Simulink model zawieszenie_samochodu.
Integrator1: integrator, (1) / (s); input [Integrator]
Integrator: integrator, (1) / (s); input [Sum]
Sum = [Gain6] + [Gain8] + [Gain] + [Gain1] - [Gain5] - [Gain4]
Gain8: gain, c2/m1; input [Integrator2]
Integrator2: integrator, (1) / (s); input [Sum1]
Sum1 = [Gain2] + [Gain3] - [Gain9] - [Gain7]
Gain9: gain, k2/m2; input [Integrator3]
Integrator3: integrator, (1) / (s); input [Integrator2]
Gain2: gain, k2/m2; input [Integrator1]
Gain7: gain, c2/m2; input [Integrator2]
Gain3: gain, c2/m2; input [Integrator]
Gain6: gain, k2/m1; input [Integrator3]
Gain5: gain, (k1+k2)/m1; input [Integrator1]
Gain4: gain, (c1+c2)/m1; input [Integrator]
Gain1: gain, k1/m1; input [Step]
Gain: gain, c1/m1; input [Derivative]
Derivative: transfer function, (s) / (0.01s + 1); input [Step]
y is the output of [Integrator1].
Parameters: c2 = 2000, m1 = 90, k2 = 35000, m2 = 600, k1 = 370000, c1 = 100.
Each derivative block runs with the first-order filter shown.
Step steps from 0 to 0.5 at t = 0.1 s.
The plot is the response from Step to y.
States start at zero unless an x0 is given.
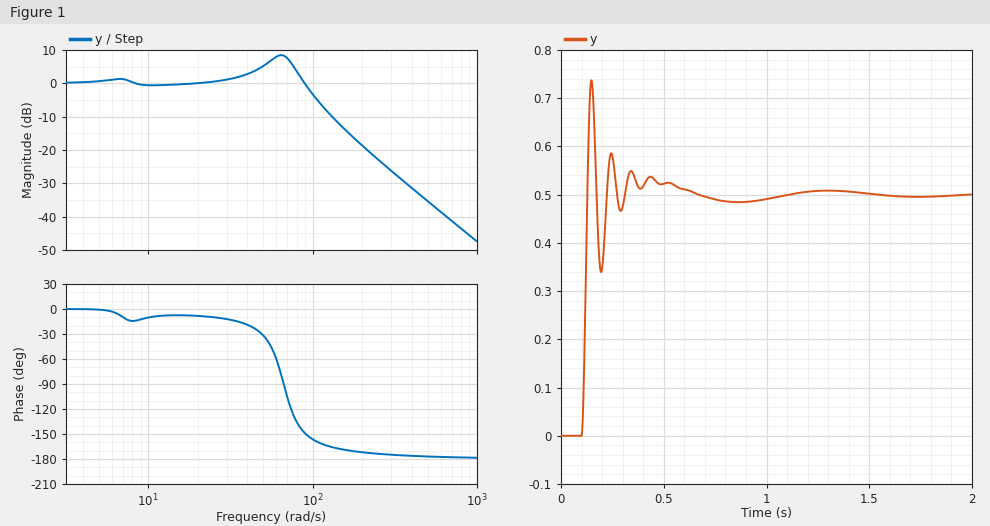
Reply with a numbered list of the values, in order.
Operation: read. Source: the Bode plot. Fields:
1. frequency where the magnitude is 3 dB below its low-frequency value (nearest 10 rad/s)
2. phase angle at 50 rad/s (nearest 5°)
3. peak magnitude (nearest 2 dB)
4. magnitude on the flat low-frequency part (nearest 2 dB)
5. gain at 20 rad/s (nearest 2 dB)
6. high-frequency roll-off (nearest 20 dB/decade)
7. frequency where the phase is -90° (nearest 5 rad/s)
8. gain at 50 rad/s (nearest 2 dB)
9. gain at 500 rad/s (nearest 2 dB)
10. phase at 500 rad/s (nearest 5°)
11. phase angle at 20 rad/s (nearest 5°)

1. 100 rad/s
2. -30°
3. 8 dB
4. 0 dB
5. 0 dB
6. -40 dB/decade
7. 65 rad/s
8. 6 dB
9. -36 dB
10. -175°
11. -10°
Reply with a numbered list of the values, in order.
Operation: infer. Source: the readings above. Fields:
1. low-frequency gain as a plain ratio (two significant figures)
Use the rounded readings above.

1. 1.0
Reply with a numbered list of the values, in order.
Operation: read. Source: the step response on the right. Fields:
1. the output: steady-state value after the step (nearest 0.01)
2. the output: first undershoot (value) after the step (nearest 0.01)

1. 0.50
2. 0.34
